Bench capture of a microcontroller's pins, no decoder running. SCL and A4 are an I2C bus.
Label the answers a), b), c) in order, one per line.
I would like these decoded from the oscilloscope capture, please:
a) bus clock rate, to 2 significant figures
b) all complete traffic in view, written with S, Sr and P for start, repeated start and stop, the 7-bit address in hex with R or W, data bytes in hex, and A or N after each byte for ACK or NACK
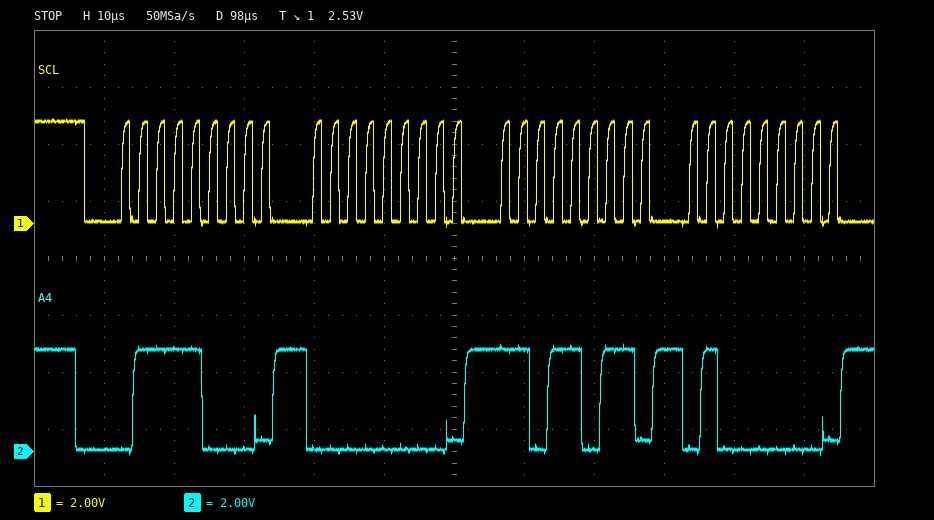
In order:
a) 400 kHz
b) S 3CW A 00 A DB A 40 A
